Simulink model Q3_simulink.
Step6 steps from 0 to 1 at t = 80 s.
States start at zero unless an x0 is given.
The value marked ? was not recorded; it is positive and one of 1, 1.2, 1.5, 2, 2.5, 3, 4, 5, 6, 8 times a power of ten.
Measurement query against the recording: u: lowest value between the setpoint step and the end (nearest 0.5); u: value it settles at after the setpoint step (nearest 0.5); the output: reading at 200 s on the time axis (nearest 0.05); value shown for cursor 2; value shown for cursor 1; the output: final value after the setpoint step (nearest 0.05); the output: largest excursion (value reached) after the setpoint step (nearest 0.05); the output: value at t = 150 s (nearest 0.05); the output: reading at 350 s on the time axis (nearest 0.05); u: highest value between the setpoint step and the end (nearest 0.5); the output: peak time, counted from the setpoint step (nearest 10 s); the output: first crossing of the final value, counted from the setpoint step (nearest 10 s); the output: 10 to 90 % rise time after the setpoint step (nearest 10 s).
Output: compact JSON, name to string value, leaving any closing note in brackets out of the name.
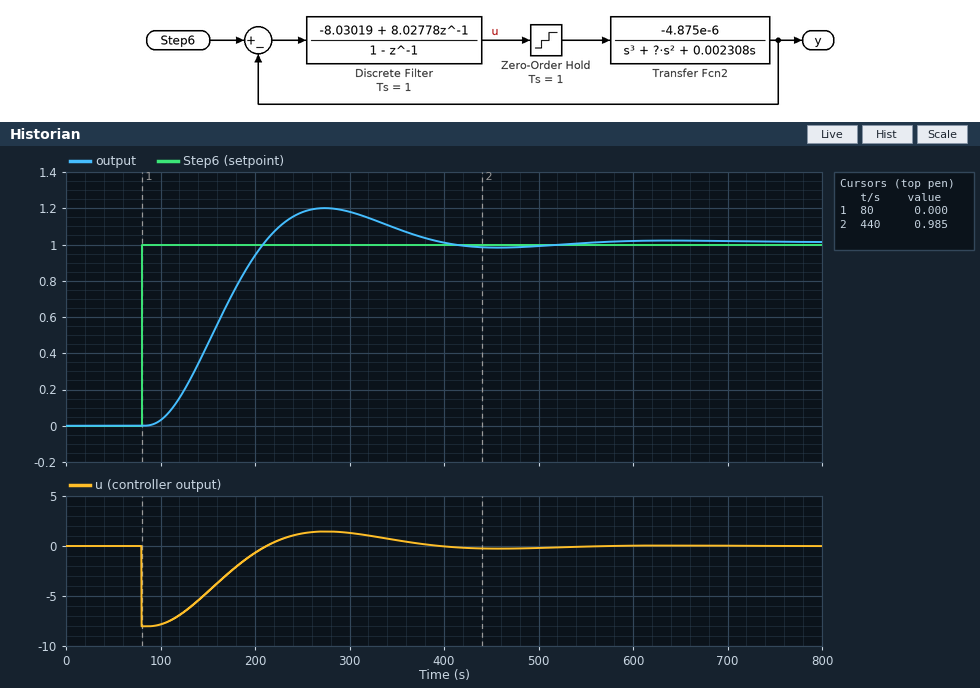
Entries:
{"u: lowest value between the setpoint step and the end": "-8.0", "u: value it settles at after the setpoint step": "0.0", "the output: reading at 200 s on the time axis": "0.95", "value shown for cursor 2": "0.985", "value shown for cursor 1": "0.000", "the output: final value after the setpoint step": "1.00", "the output: largest excursion (value reached) after the setpoint step": "1.20", "the output: value at t = 150 s": "0.45", "the output: reading at 350 s on the time axis": "1.10", "u: highest value between the setpoint step and the end": "1.5", "the output: peak time, counted from the setpoint step": "190 s", "the output: first crossing of the final value, counted from the setpoint step": "130 s", "the output: 10 to 90 % rise time after the setpoint step": "80 s"}
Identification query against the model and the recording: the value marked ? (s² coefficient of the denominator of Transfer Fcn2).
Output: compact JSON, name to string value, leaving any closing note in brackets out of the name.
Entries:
{"the value marked ?": "0.12"}
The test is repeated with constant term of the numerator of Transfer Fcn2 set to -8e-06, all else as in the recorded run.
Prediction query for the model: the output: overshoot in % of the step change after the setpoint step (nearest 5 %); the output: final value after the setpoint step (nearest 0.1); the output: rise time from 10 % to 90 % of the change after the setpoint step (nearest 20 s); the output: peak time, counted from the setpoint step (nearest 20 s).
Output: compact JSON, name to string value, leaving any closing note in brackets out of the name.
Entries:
{"the output: overshoot in % of the step change after the setpoint step": "35 %", "the output: final value after the setpoint step": "1.0", "the output: rise time from 10 % to 90 % of the change after the setpoint step": "60 s", "the output: peak time, counted from the setpoint step": "140 s"}
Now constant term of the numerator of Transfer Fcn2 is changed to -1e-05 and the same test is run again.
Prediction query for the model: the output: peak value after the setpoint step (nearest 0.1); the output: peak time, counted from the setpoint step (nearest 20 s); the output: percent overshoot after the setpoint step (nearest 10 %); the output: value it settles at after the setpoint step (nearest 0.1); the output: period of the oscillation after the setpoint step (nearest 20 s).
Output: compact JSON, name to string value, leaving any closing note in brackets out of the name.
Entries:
{"the output: peak value after the setpoint step": "1.4", "the output: peak time, counted from the setpoint step": "120 s", "the output: percent overshoot after the setpoint step": "40 %", "the output: value it settles at after the setpoint step": "1.0", "the output: period of the oscillation after the setpoint step": "240 s"}
